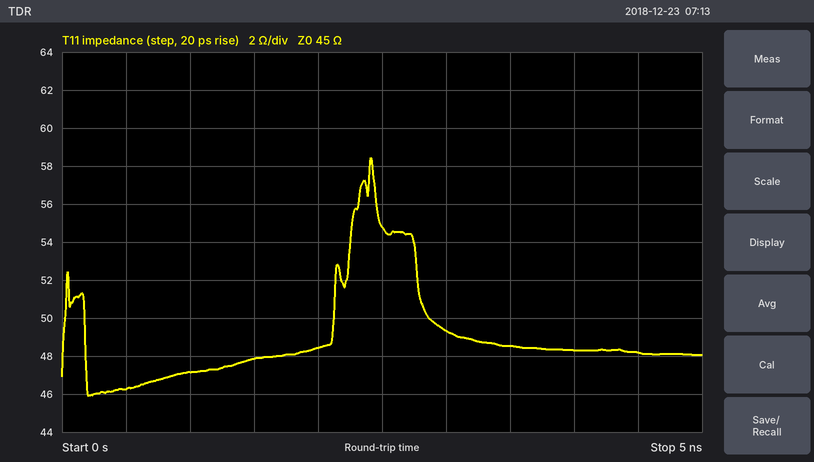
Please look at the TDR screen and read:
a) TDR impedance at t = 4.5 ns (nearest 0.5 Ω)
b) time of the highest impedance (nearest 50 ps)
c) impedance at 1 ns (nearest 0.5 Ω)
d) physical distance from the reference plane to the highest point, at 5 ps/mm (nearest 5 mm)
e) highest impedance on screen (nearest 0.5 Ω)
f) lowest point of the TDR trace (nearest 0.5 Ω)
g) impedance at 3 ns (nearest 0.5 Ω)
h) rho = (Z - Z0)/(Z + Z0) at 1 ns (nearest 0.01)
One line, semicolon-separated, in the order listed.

48.0 Ω; 2.40 ns; 47.0 Ω; 240 mm; 58.5 Ω; 46.0 Ω; 49.5 Ω; +0.02
